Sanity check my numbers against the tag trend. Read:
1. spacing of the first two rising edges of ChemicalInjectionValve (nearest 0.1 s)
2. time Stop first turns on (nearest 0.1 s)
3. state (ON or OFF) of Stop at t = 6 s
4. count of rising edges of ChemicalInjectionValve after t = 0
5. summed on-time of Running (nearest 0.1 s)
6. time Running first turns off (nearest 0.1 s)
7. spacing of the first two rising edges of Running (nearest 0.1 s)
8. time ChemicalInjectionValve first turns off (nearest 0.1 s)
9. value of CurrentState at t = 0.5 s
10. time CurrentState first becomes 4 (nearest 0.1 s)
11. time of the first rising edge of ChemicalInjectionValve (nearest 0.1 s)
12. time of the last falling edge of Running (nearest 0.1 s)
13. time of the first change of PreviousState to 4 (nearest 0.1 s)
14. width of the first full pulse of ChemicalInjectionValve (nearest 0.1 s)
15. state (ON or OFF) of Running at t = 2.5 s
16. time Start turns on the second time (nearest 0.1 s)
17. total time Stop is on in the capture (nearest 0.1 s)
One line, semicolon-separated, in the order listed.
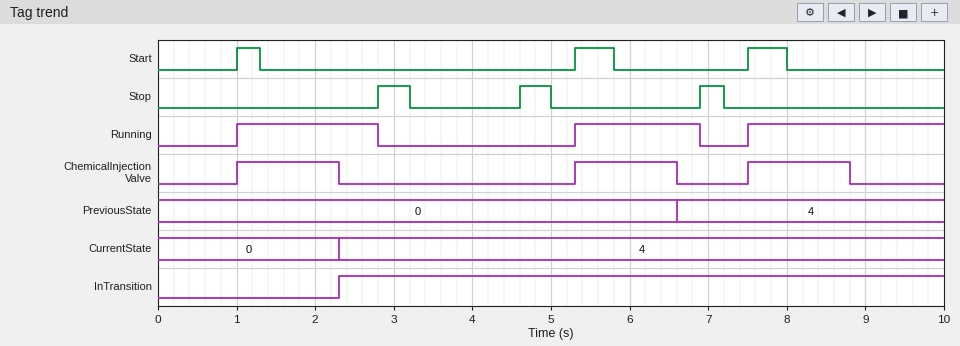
4.3 s; 2.8 s; OFF; 3; 5.9 s; 2.8 s; 4.3 s; 2.3 s; 0; 2.3 s; 1.0 s; 6.9 s; 6.6 s; 1.3 s; ON; 5.3 s; 1.1 s
